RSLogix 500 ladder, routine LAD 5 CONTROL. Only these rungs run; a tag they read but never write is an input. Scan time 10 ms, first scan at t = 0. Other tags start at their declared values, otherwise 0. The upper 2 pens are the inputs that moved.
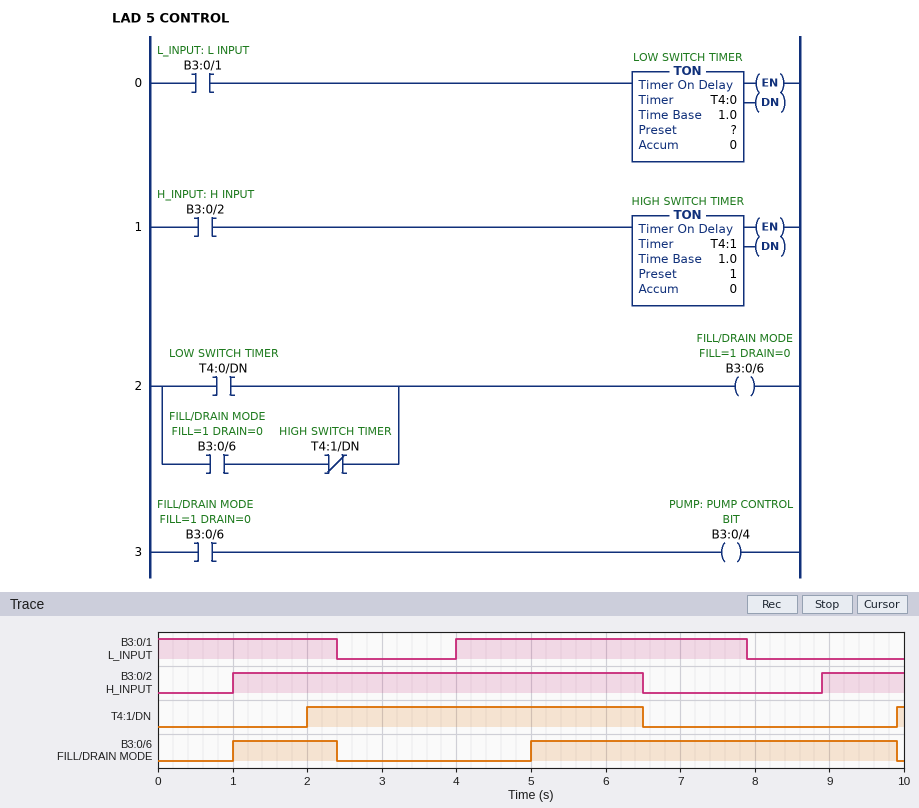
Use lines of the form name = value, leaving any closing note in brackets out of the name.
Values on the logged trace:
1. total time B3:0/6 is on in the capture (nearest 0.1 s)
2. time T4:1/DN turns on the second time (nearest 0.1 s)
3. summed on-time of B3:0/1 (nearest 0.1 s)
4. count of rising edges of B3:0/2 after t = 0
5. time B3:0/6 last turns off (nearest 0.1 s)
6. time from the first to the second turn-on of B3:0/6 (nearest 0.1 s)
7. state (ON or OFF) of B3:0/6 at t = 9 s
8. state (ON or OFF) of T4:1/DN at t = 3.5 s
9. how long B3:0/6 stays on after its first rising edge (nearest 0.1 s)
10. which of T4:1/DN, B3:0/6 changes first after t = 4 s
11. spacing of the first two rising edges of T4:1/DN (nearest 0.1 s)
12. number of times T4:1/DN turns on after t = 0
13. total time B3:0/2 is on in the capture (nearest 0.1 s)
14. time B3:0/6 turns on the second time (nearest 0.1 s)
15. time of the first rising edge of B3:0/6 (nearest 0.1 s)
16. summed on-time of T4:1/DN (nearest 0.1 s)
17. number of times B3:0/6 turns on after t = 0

total time B3:0/6 is on in the capture = 6.3 s
time T4:1/DN turns on the second time = 9.9 s
summed on-time of B3:0/1 = 6.3 s
count of rising edges of B3:0/2 after t = 0 = 2
time B3:0/6 last turns off = 9.9 s
time from the first to the second turn-on of B3:0/6 = 4.0 s
state (ON or OFF) of B3:0/6 at t = 9 s = ON
state (ON or OFF) of T4:1/DN at t = 3.5 s = ON
how long B3:0/6 stays on after its first rising edge = 1.4 s
which of T4:1/DN, B3:0/6 changes first after t = 4 s = B3:0/6
spacing of the first two rising edges of T4:1/DN = 7.9 s
number of times T4:1/DN turns on after t = 0 = 2
total time B3:0/2 is on in the capture = 6.6 s
time B3:0/6 turns on the second time = 5.0 s
time of the first rising edge of B3:0/6 = 1.0 s
summed on-time of T4:1/DN = 4.6 s
number of times B3:0/6 turns on after t = 0 = 2
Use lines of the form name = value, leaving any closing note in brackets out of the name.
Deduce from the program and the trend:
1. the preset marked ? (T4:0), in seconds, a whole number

the preset marked ? (T4:0), in seconds, a whole number = 1 s
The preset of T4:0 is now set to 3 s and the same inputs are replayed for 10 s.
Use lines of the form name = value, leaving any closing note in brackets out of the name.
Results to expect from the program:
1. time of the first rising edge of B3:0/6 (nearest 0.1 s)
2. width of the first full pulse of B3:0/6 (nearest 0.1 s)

time of the first rising edge of B3:0/6 = 7.0 s
width of the first full pulse of B3:0/6 = 2.9 s
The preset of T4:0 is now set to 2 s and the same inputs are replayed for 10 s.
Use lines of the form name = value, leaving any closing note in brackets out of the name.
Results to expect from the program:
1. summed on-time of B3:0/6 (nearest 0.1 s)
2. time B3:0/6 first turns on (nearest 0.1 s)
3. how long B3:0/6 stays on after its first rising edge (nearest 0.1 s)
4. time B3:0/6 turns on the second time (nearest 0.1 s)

summed on-time of B3:0/6 = 4.3 s
time B3:0/6 first turns on = 2.0 s
how long B3:0/6 stays on after its first rising edge = 0.4 s
time B3:0/6 turns on the second time = 6.0 s
